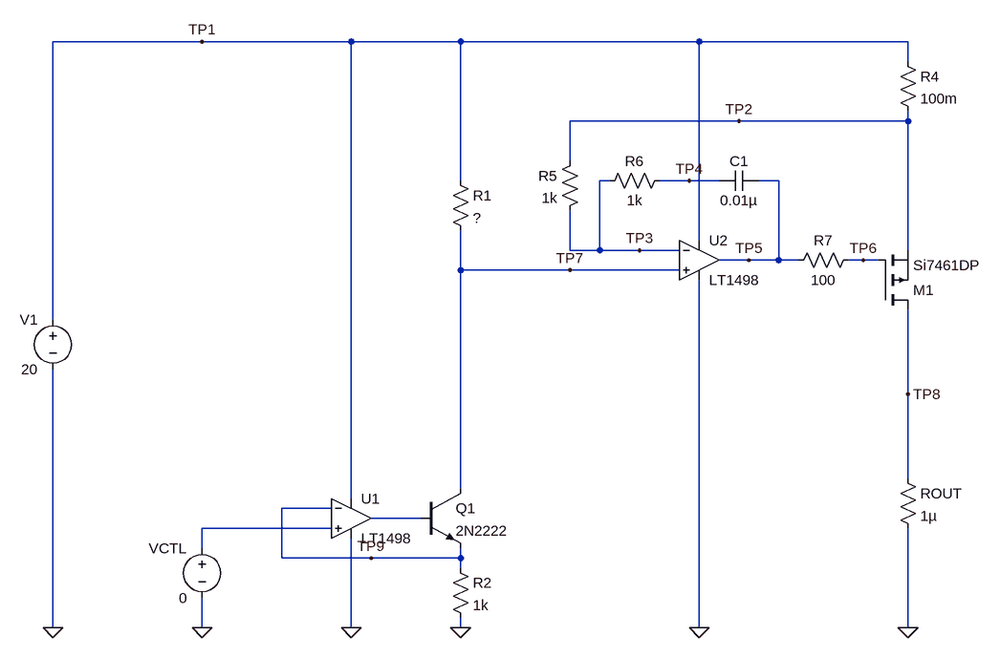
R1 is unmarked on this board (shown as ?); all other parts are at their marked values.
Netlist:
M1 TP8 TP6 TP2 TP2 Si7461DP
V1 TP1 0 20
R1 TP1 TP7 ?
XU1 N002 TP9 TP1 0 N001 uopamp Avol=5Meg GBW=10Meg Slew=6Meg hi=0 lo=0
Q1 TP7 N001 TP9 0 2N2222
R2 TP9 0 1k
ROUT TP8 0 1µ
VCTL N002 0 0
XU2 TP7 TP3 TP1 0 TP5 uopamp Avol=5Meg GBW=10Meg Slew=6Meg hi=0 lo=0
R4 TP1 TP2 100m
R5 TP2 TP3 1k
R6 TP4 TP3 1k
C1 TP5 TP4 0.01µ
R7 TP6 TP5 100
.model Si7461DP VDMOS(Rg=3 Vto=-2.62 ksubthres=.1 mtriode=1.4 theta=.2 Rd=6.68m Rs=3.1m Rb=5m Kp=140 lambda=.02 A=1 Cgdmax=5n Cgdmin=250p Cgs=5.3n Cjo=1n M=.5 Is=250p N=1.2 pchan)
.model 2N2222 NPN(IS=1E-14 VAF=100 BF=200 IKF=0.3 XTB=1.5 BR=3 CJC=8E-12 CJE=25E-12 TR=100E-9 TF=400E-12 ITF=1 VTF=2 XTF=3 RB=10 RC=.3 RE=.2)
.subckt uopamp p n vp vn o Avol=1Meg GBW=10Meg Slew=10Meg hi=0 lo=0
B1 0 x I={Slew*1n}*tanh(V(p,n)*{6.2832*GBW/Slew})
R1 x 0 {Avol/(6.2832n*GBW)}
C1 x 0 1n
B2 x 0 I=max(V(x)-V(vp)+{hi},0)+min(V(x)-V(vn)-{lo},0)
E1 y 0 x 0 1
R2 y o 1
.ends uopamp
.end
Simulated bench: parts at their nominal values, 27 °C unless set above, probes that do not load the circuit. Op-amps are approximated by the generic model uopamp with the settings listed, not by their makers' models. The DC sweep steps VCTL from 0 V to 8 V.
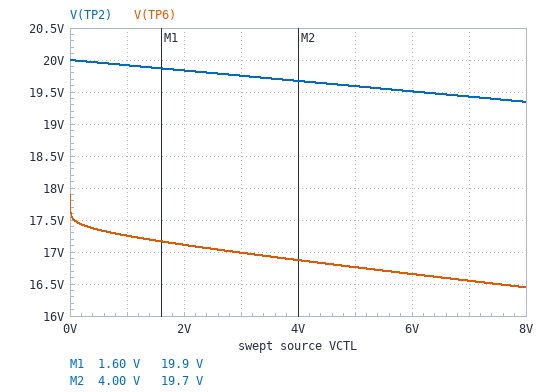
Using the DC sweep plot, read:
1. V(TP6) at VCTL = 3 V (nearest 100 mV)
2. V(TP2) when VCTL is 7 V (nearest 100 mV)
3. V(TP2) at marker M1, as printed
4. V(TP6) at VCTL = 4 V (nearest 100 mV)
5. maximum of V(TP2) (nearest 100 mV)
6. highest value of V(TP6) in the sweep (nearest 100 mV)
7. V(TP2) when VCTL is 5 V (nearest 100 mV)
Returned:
17.0 V
19.4 V
19.9 V
16.9 V
20.0 V
17.9 V
19.6 V
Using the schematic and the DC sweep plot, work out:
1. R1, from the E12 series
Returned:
82 Ω
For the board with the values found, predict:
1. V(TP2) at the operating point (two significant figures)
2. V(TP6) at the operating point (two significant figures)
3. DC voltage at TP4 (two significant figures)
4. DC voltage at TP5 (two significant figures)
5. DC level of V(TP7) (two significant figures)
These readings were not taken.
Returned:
20 V
18 V
20 V
18 V
20 V
